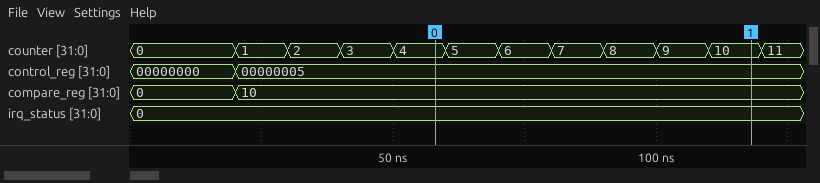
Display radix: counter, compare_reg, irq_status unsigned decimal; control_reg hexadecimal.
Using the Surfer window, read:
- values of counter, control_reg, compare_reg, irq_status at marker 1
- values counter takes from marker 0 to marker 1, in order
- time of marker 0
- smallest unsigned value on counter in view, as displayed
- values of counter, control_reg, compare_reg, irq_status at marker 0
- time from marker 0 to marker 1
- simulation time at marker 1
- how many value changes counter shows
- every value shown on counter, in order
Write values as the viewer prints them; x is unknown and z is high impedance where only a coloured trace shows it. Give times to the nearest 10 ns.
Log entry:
counter=10, control_reg=00000005, compare_reg=10, irq_status=0
4, 5, 6, 7, 8, 9, 10
60 ns
0
counter=4, control_reg=00000005, compare_reg=10, irq_status=0
60 ns
120 ns
11
0, 1, 2, 3, 4, 5, 6, 7, 8, 9, 10, 11
